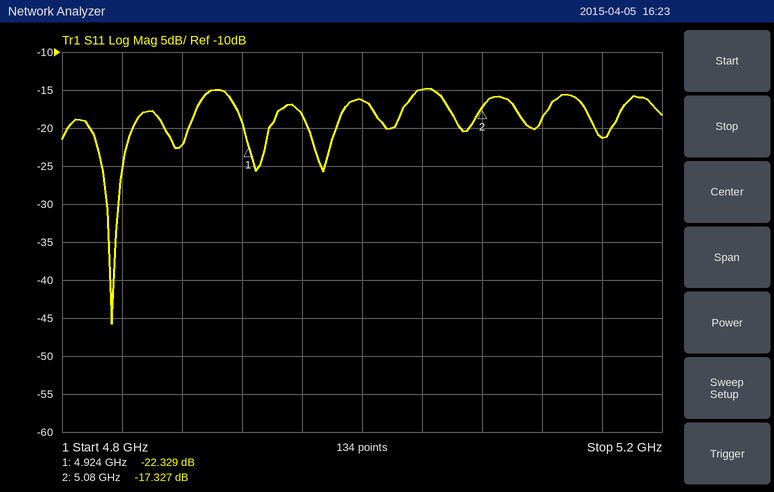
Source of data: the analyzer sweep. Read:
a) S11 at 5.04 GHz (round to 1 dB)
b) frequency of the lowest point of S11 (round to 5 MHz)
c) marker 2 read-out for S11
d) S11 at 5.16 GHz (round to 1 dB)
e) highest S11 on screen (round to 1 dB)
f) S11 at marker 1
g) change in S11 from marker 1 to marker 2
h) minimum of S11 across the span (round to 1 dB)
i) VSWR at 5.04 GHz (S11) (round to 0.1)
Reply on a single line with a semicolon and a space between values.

-15 dB; 4.835 GHz; -17.327 dB; -21 dB; -15 dB; -22.329 dB; 5.002 dB; -46 dB; 1.4
